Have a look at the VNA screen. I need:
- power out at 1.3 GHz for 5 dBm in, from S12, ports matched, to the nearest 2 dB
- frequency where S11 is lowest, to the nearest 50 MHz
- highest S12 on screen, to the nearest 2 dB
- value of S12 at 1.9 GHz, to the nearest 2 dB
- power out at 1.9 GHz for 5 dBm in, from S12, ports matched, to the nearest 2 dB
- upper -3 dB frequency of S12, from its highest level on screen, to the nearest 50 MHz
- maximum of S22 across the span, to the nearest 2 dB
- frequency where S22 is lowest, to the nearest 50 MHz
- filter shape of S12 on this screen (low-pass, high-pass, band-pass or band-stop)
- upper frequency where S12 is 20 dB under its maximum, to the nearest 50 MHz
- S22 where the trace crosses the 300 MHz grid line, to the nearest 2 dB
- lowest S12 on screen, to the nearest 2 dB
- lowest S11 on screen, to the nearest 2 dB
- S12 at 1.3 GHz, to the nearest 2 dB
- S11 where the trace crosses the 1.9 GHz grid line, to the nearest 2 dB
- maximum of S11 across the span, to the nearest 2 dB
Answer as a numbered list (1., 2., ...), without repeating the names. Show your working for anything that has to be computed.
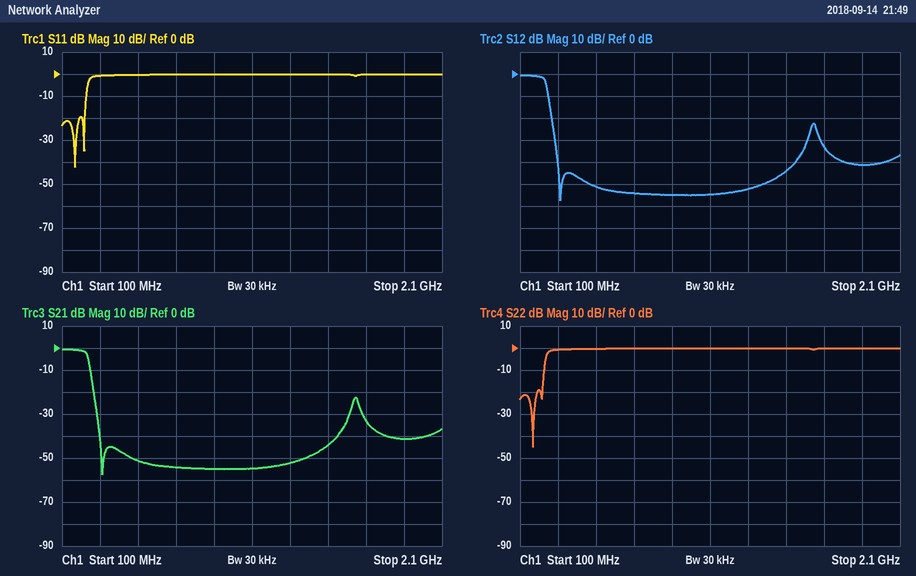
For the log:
1. 5 dBm + (-52 dB) = -48 dBm
2. 150 MHz
3. 0 dB
4. -42 dB
5. 5 dBm + (-42 dB) = -36 dBm
6. 250 MHz
7. 0 dB
8. 150 MHz
9. low-pass
10. 250 MHz
11. 0 dB
12. -58 dB
13. -42 dB
14. -52 dB
15. 0 dB
16. 0 dB
